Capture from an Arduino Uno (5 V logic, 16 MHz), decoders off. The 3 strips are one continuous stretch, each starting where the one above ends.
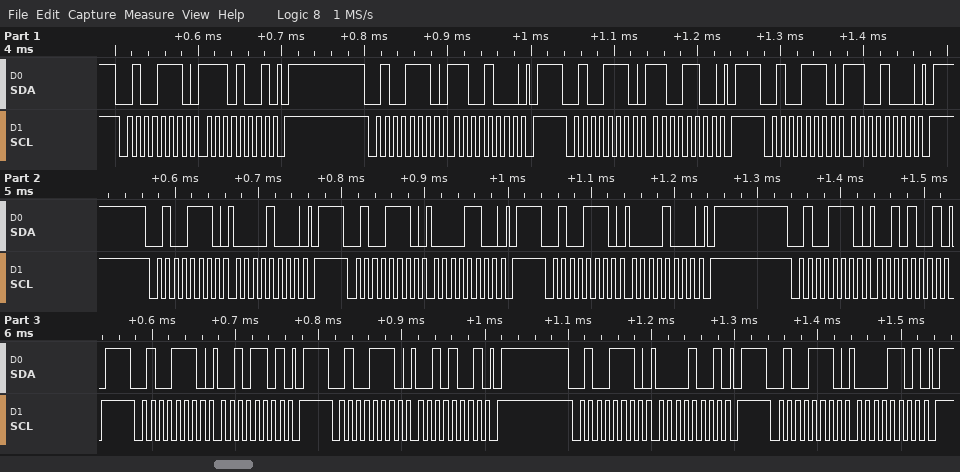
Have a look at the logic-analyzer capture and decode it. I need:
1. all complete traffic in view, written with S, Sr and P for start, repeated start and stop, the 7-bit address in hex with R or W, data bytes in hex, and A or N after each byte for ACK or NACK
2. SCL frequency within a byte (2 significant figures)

S 27W A E9 A P S 27W A C8 A P S 27W A CC A P S 27W A C8 A P S 27W A 08 A P S 27W A 0C A P S 27W A 08 A P S 27W A 29 A P S 27W A 2D A P S 27W A 29 A P S 27W A 09 A P S 27W A 0D A P
100 kHz
